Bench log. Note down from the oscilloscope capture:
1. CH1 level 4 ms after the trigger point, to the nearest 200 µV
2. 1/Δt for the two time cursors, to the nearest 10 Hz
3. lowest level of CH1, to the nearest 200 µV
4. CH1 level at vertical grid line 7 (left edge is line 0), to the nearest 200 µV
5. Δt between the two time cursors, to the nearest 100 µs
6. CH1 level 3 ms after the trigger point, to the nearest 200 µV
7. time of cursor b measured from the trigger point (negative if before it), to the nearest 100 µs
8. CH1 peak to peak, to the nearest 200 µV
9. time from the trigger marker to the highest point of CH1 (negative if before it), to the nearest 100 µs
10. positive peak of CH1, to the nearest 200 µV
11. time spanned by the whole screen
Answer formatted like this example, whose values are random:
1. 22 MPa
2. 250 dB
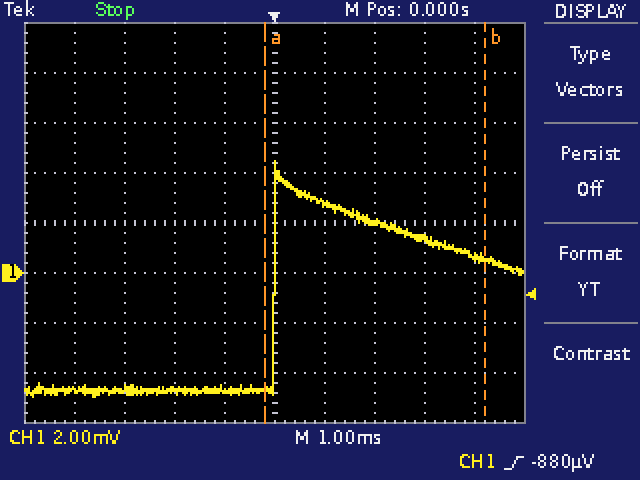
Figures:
1. 600 µV
2. 230 Hz
3. -5.0 mV
4. 2.0 mV
5. 4.4 ms
6. 1.4 mV
7. +4.2 ms
8. 9.4 mV
9. 0.0 ms
10. 4.4 mV
11. 10 ms
